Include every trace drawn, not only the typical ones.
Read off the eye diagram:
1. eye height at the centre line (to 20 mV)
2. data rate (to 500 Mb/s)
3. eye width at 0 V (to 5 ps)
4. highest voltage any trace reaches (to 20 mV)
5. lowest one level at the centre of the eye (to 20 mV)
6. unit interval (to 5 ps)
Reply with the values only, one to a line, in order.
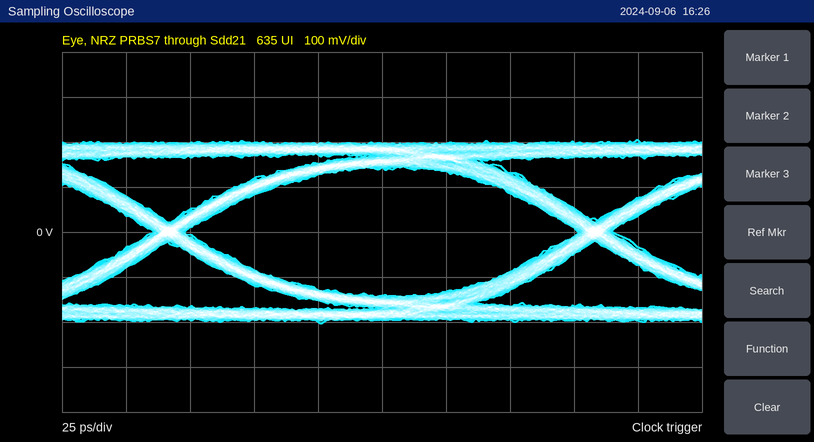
280 mV
6.0 Gb/s
155 ps
200 mV
140 mV
165 ps
